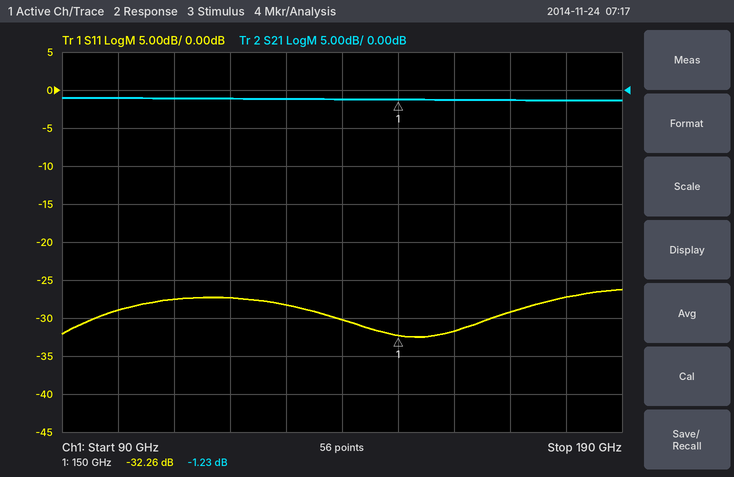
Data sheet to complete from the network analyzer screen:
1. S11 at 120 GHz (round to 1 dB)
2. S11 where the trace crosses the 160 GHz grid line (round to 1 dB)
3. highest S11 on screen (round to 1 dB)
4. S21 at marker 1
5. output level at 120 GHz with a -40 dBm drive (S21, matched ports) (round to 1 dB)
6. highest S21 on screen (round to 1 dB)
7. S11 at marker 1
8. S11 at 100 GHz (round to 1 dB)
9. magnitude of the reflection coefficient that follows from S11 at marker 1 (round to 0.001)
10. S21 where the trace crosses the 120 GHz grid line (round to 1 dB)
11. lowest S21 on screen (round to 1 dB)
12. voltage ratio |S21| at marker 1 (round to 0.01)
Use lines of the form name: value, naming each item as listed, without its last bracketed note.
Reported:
S11 at 120 GHz: -27 dB
S11 where the trace crosses the 160 GHz grid line: -32 dB
highest S11 on screen: -26 dB
S21 at marker 1: -1.23 dB
output level at 120 GHz with a -40 dBm drive (S21, matched ports): -41 dBm
highest S21 on screen: -1 dB
S11 at marker 1: -32.26 dB
S11 at 100 GHz: -29 dB
magnitude of the reflection coefficient that follows from S11 at marker 1: 0.024
S21 where the trace crosses the 120 GHz grid line: -1 dB
lowest S21 on screen: -1 dB
voltage ratio |S21| at marker 1: 0.87
